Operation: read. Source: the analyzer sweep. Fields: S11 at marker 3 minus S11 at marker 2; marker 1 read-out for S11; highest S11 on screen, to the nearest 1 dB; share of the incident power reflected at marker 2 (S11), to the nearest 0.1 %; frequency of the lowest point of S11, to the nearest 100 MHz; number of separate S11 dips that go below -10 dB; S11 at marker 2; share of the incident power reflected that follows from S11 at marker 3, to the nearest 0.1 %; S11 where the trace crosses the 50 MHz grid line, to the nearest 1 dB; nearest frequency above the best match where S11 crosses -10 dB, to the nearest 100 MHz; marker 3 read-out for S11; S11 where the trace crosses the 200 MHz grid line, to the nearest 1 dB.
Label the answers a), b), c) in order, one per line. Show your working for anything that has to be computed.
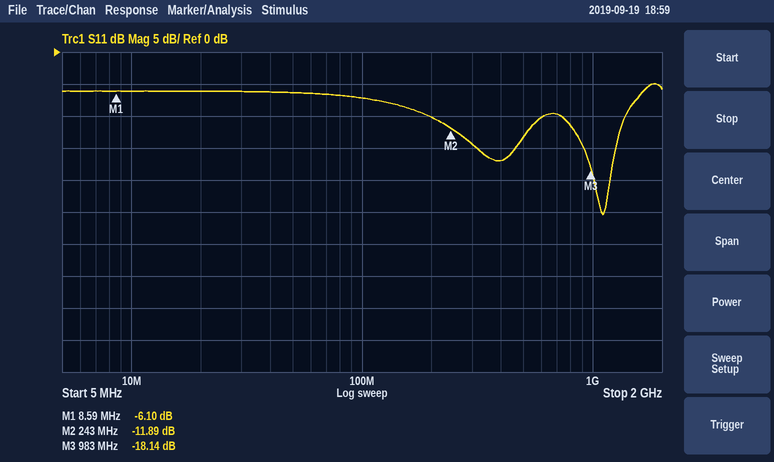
a) -18.14 − (-11.89) = -6.25 dB
b) -6.10 dB
c) -5 dB
d) 10^(-11.89/10) ≈ 6.5 %
e) 1.1 GHz
f) 2
g) -11.89 dB
h) 10^(-18.14/10) ≈ 1.5 %
i) -6 dB
j) 1.4 GHz
k) -18.14 dB
l) -10 dB
